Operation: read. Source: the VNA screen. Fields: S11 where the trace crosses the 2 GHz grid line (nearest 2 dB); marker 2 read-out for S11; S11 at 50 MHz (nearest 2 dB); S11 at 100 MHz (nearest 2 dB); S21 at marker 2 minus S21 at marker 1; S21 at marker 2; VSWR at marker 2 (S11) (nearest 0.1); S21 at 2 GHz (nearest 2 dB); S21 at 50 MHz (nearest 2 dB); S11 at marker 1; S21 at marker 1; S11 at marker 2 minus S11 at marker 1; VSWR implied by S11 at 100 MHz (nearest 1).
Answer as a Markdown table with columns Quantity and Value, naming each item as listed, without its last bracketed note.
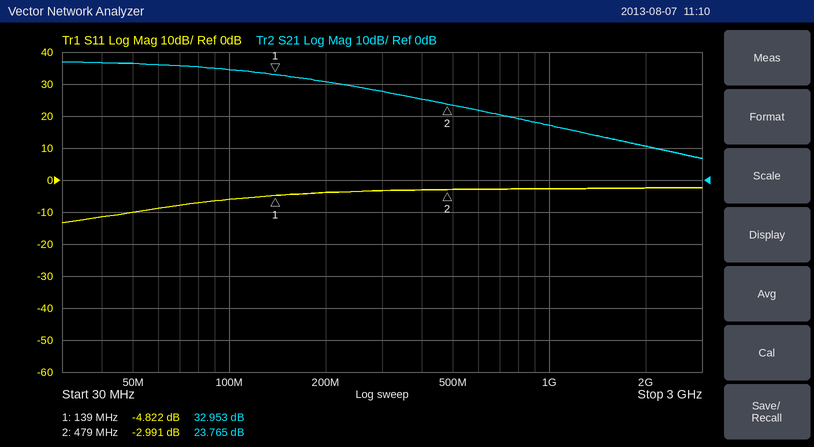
| Quantity | Value |
|---|---|
| S11 where the trace crosses the 2 GHz grid line | -2 dB |
| marker 2 read-out for S11 | -2.991 dB |
| S11 at 50 MHz | -10 dB |
| S11 at 100 MHz | -6 dB |
| S21 at marker 2 minus S21 at marker 1 | -9.188 dB |
| S21 at marker 2 | 23.765 dB |
| VSWR at marker 2 (S11) | 5.9 |
| S21 at 2 GHz | 10 dB |
| S21 at 50 MHz | 36 dB |
| S11 at marker 1 | -4.822 dB |
| S21 at marker 1 | 32.953 dB |
| S11 at marker 2 minus S11 at marker 1 | 1.831 dB |
| VSWR implied by S11 at 100 MHz | 3 |
